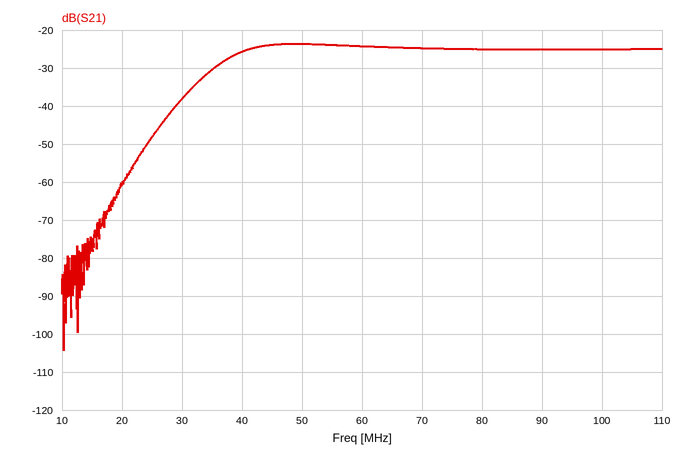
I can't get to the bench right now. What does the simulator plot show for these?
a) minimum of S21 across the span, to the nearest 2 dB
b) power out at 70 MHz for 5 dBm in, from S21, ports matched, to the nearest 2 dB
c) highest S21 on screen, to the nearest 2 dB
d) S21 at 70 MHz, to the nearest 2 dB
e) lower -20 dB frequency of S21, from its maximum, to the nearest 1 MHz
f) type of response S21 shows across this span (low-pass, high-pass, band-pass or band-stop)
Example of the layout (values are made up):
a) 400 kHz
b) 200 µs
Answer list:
a) -104 dB
b) -20 dBm
c) -24 dB
d) -24 dB
e) 27 MHz
f) high-pass
